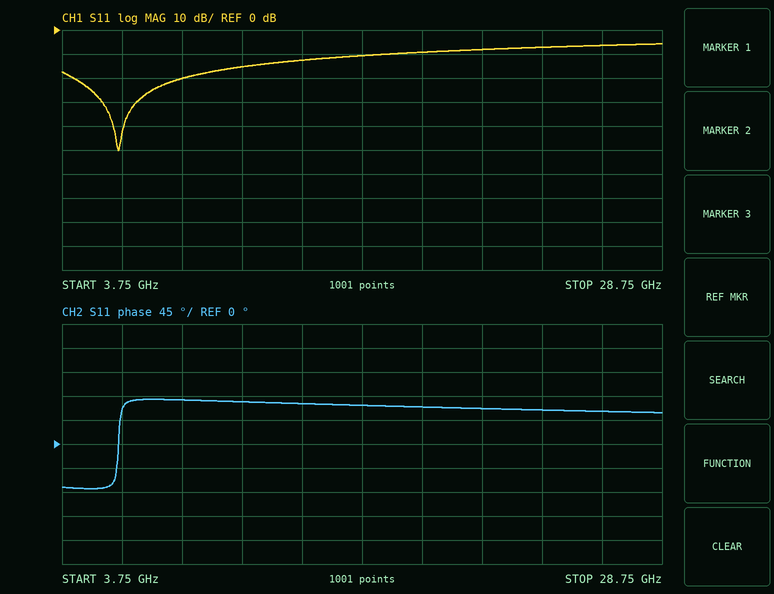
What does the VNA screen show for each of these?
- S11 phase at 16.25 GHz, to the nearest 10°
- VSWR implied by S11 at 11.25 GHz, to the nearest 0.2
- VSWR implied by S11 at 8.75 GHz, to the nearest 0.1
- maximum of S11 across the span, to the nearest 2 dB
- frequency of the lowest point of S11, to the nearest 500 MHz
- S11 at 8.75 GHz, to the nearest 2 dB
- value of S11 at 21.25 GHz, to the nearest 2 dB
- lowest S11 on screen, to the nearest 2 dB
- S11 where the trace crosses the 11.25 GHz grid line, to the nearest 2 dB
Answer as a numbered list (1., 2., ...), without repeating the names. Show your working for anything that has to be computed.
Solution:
1. 70°
2. |Γ| = 10^(-16/20) = 0.1585; VSWR = (1 + 0.1585)/(1 − 0.1585) ≈ 1.4
3. |Γ| = 10^(-20/20) = 0.1000; VSWR = (1 + 0.1000)/(1 − 0.1000) ≈ 1.2
4. -6 dB
5. 6.0 GHz
6. -20 dB
7. -8 dB
8. -50 dB
9. -16 dB
